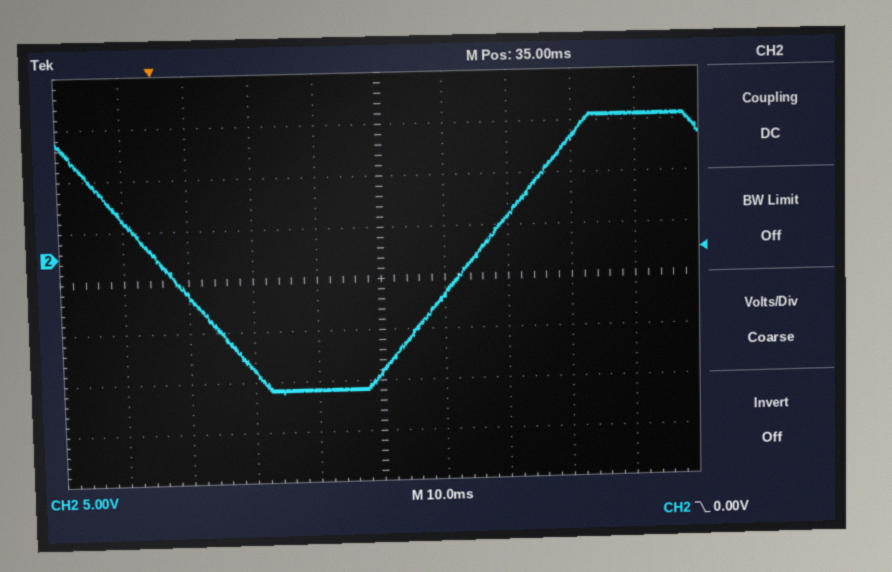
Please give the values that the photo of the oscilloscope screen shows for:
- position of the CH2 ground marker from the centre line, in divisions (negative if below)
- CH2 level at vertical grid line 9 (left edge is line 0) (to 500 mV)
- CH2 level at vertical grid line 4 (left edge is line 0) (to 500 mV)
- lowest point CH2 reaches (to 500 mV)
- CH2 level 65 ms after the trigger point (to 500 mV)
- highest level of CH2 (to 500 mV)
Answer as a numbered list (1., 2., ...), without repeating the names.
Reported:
1. +0.5 div
2. 13.0 V
3. -13.5 V
4. -13.5 V
5. 11.0 V
6. 13.0 V
